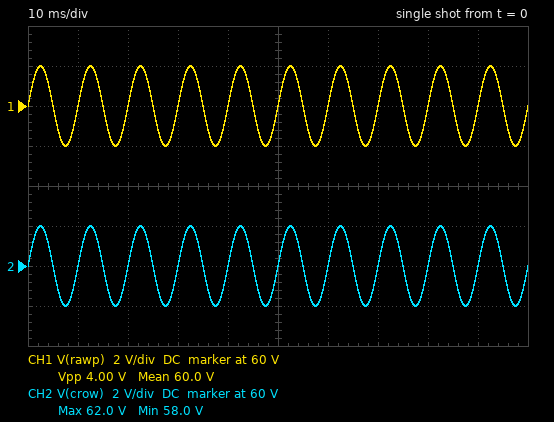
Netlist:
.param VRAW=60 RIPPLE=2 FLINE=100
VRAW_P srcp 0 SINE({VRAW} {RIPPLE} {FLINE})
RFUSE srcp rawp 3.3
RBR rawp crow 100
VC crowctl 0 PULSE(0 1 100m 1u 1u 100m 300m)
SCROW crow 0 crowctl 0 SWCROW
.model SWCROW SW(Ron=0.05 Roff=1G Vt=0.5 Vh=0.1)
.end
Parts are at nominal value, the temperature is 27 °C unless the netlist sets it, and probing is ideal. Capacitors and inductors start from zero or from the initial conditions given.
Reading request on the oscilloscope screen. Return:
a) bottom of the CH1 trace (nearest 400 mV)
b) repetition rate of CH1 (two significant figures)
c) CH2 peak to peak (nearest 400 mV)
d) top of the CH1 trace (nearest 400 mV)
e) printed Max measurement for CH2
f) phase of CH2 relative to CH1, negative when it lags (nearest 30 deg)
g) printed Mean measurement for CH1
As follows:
58.0 V
100 Hz
4.0 V
62.0 V
62.0 V
0 deg
60.0 V
